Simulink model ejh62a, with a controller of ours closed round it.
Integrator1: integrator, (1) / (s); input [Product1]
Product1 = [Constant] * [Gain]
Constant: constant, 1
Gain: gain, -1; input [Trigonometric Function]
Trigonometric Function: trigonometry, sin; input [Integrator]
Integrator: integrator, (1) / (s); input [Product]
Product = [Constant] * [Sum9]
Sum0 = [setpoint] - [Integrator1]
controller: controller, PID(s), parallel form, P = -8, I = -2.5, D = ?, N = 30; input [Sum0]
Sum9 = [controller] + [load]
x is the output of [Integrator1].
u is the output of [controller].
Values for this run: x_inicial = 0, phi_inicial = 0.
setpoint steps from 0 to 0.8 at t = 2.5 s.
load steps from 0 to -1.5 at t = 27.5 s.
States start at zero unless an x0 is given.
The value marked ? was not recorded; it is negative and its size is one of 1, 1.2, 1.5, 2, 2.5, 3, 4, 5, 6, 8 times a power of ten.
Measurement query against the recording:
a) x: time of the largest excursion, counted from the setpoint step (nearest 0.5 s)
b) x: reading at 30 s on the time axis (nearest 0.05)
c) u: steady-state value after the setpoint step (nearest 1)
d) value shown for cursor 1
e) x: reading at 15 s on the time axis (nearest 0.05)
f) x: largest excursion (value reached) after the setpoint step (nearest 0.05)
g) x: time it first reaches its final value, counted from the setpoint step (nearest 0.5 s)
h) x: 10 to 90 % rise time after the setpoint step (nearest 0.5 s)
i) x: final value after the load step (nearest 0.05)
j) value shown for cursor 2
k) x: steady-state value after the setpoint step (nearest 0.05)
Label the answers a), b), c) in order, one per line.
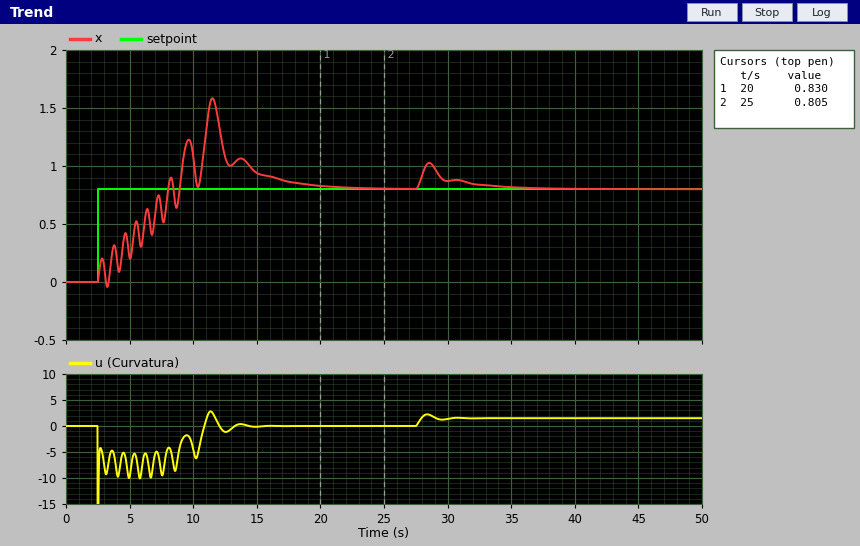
a) 9.0 s
b) 0.85
c) 0
d) 0.830
e) 0.95
f) 1.60
g) 5.5 s
h) 4.5 s
i) 0.80
j) 0.805
k) 0.80
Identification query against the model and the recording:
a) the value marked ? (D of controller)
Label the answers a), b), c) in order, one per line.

a) -2
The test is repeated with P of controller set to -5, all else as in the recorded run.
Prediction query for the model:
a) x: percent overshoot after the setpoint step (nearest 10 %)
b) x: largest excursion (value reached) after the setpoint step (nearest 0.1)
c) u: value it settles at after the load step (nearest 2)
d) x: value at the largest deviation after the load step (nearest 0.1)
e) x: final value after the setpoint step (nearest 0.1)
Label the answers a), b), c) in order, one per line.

a) 110 %
b) 1.7
c) 2
d) 1.1
e) 0.8
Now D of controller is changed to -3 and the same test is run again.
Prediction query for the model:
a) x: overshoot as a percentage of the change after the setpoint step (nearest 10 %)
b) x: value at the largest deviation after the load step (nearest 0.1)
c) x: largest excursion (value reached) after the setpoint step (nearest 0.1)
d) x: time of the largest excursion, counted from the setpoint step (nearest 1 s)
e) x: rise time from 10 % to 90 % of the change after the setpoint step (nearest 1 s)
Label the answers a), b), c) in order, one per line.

a) 60 %
b) 1.0
c) 1.3
d) 7 s
e) 4 s
